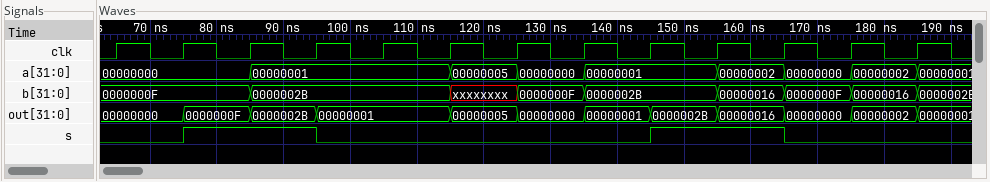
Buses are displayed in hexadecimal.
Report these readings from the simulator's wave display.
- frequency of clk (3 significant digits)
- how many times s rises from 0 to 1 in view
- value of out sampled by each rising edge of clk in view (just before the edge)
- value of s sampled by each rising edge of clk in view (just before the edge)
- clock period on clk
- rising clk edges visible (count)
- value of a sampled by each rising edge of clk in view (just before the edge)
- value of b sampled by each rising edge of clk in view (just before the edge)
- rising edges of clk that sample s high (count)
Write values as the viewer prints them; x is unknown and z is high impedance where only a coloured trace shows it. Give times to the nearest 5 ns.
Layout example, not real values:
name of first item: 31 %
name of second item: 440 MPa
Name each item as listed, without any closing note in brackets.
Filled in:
frequency of clk: 100 MHz
how many times s rises from 0 to 1 in view: 2
value of out sampled by each rising edge of clk in view: 00000000, 00000000, 0000000F, 0000002B, 00000001, 00000001, 00000005, 00000000, 00000001, 0000002B, 00000016, 00000000, 00000002
value of s sampled by each rising edge of clk in view: 0 0 1 1 0 0 0 0 0 1 1 0 0
clock period on clk: 10 ns
rising clk edges visible: 13
value of a sampled by each rising edge of clk in view: 00000000, 00000000, 00000000, 00000001, 00000001, 00000001, 00000005, 00000000, 00000001, 00000001, 00000002, 00000000, 00000002
value of b sampled by each rising edge of clk in view: 0000000F, 0000000F, 0000000F, 0000002B, 0000002B, 0000002B, xxxxxxxx, 0000000F, 0000002B, 0000002B, 00000016, 0000000F, 00000016
rising edges of clk that sample s high: 4
